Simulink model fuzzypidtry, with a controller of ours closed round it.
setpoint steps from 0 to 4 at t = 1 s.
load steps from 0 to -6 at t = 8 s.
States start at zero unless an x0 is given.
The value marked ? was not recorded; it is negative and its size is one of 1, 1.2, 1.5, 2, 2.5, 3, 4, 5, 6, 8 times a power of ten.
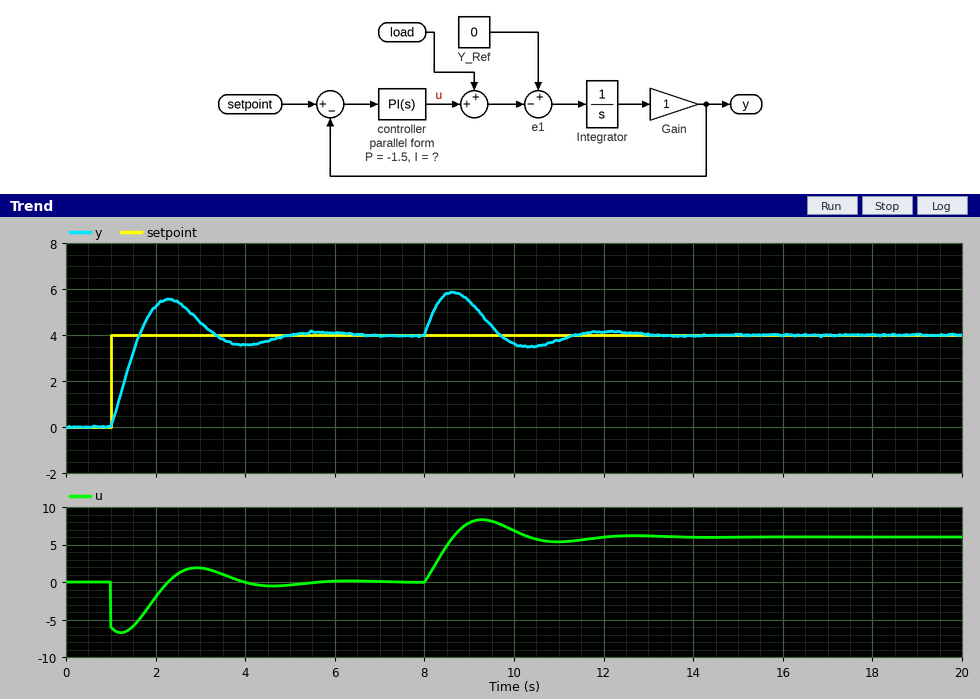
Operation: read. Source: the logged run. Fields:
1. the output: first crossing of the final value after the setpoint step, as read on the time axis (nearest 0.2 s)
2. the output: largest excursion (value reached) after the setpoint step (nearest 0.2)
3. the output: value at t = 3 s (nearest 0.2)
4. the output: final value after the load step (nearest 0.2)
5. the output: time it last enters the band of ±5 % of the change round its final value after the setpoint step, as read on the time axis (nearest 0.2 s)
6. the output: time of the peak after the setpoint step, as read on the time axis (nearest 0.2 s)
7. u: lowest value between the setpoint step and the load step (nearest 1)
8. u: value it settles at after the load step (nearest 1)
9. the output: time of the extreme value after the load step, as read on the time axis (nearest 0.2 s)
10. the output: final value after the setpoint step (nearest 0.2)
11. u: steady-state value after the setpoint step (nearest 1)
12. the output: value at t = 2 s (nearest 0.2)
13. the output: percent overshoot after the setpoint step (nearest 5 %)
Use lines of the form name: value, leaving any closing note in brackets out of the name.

the output: first crossing of the final value after the setpoint step, as read on the time axis: 1.6 s
the output: largest excursion (value reached) after the setpoint step: 5.6
the output: value at t = 3 s: 4.6
the output: final value after the load step: 4.0
the output: time it last enters the band of ±5 % of the change round its final value after the setpoint step, as read on the time axis: 4.6 s
the output: time of the peak after the setpoint step, as read on the time axis: 2.2 s
u: lowest value between the setpoint step and the load step: -7
u: value it settles at after the load step: 6
the output: time of the extreme value after the load step, as read on the time axis: 8.6 s
the output: final value after the setpoint step: 4.0
u: steady-state value after the setpoint step: 0
the output: value at t = 2 s: 5.2
the output: percent overshoot after the setpoint step: 40 %
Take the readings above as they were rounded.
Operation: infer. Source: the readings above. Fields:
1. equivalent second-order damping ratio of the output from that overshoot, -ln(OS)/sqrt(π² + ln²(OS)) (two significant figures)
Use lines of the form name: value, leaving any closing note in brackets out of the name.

equivalent second-order damping ratio of the output from that overshoot, -ln(OS)/sqrt(π² + ln²(OS)): 0.28
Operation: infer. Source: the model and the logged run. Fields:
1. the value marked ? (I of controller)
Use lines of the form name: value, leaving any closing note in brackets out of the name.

the value marked ?: -4
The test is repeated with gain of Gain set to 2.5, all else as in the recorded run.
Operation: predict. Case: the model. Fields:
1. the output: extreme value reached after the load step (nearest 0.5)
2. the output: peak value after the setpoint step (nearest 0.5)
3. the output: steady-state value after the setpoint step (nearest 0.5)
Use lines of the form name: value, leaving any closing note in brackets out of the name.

the output: extreme value reached after the load step: 6.5
the output: peak value after the setpoint step: 5.0
the output: steady-state value after the setpoint step: 4.0
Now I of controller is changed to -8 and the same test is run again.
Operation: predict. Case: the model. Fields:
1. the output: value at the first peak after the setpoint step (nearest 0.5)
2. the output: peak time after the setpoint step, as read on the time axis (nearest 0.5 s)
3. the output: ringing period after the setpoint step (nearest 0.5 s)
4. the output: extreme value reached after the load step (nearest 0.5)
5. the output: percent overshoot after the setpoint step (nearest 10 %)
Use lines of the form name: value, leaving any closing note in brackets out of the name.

the output: value at the first peak after the setpoint step: 6.0
the output: peak time after the setpoint step, as read on the time axis: 2.0 s
the output: ringing period after the setpoint step: 2.5 s
the output: extreme value reached after the load step: 5.5
the output: percent overshoot after the setpoint step: 50 %
